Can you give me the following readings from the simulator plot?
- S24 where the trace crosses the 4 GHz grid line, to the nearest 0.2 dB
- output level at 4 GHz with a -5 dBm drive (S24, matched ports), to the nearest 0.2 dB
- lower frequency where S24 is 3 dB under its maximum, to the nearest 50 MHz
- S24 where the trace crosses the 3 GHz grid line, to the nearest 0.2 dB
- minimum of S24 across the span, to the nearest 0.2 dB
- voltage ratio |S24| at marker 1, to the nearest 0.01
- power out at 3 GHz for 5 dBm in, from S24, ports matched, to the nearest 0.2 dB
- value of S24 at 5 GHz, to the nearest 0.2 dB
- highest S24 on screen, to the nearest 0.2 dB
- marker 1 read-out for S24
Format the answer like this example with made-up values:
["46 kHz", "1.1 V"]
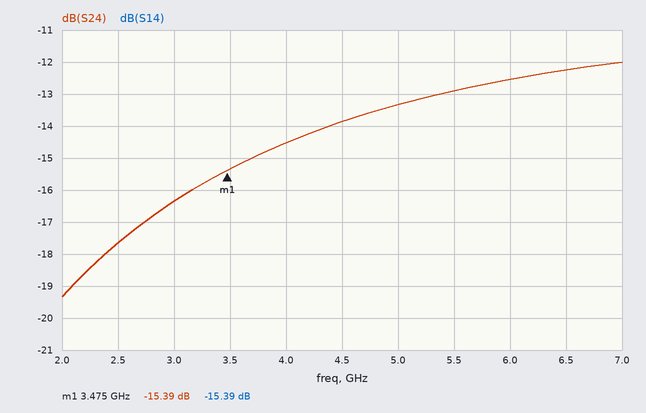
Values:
["-14.6 dB", "-19.6 dBm", "3.70 GHz", "-16.4 dB", "-19.4 dB", "0.17", "-11.4 dBm", "-13.4 dB", "-12.0 dB", "-15.39 dB"]
